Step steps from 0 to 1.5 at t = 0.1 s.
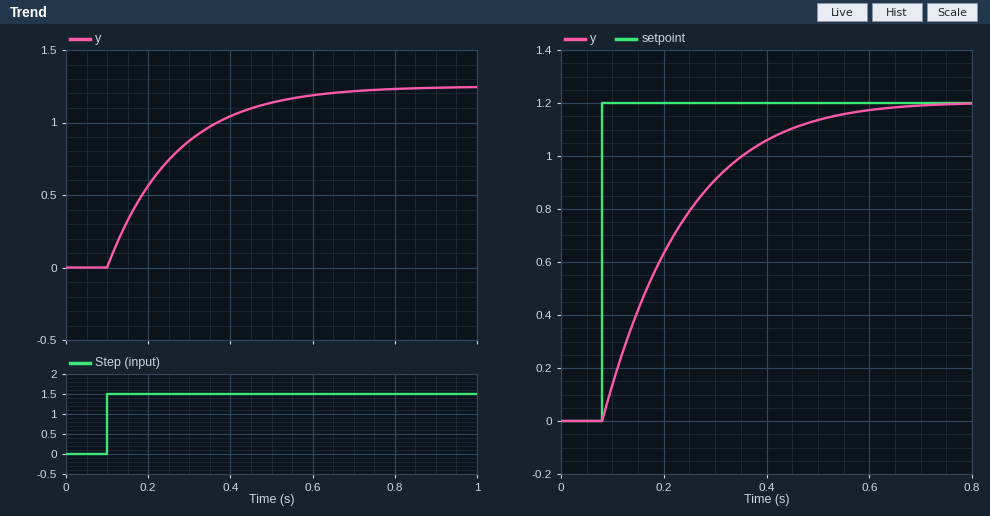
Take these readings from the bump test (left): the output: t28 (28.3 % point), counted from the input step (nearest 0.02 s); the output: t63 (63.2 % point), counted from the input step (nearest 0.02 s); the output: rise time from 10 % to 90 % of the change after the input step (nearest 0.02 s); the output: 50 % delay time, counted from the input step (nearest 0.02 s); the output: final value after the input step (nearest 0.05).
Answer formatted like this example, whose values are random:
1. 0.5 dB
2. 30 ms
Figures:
1. 0.06 s
2. 0.16 s
3. 0.36 s
4. 0.12 s
5. 1.25
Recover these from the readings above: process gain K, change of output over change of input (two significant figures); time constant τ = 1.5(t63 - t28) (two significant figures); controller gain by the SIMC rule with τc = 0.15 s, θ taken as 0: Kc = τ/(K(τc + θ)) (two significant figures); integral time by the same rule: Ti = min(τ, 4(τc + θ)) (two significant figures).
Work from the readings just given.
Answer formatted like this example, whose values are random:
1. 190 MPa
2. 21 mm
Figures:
1. 0.83
2. 0.15 s
3. 1.2
4. 0.15 s
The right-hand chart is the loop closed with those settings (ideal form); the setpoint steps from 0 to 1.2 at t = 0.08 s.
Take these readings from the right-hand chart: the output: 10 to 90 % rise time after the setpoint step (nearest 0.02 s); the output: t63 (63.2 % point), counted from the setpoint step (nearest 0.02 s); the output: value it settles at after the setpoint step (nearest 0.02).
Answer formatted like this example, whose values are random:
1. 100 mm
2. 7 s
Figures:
1. 0.32 s
2. 0.16 s
3. 1.20
